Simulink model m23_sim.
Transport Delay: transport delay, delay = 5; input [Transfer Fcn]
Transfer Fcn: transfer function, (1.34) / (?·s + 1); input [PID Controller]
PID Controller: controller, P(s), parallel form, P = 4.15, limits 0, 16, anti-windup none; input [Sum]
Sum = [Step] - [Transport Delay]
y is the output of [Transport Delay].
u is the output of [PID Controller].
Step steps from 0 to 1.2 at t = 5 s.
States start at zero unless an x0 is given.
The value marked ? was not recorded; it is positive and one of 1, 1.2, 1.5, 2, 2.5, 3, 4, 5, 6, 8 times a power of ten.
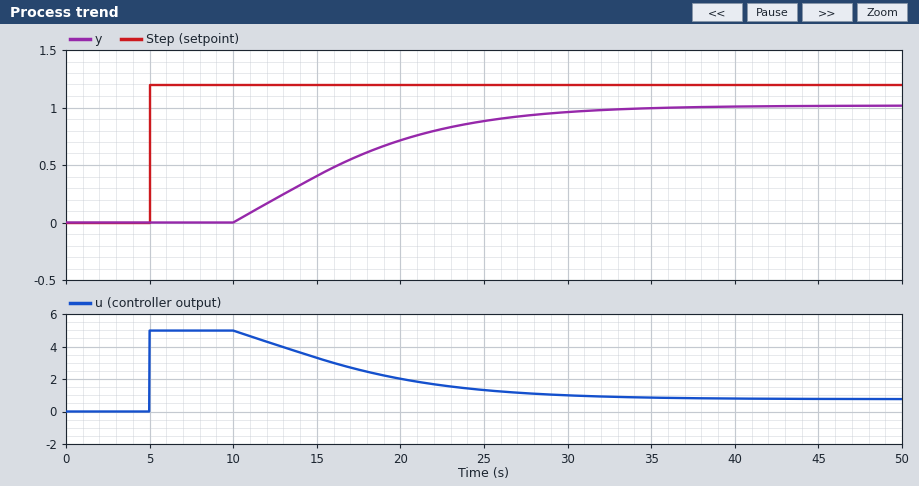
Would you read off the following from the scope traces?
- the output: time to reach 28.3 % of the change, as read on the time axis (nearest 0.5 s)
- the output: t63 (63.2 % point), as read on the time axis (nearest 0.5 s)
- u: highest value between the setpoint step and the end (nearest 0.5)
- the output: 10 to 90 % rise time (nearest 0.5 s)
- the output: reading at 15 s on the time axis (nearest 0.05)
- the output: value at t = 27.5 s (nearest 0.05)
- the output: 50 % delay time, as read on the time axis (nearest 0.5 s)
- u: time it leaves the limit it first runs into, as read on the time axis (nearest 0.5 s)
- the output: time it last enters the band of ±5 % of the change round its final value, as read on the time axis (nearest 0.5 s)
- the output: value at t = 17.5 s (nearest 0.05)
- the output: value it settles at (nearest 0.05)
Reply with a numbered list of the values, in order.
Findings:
1. 13.5 s
2. 18.5 s
3. 5.0
4. 15.5 s
5. 0.40
6. 0.95
7. 16.5 s
8. 10.0 s
9. 30.5 s
10. 0.60
11. 1.00
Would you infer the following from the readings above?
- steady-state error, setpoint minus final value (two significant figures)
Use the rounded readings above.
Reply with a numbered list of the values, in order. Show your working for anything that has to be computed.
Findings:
1. 1.2 - 1 = 0.20
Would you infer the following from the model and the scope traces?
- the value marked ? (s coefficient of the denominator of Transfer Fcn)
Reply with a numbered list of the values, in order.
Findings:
1. 80
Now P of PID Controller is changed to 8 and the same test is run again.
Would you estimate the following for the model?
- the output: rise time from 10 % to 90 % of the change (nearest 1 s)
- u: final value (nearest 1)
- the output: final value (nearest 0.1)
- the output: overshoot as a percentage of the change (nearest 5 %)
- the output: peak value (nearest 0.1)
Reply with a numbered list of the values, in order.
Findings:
1. 6 s
2. 1
3. 1.1
4. 20 %
5. 1.3
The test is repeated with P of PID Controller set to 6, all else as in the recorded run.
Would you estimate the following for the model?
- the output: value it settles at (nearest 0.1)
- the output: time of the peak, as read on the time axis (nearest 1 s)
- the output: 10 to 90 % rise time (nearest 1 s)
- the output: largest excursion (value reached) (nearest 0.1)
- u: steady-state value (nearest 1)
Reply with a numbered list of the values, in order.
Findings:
1. 1.1
2. 27 s
3. 9 s
4. 1.1
5. 1
